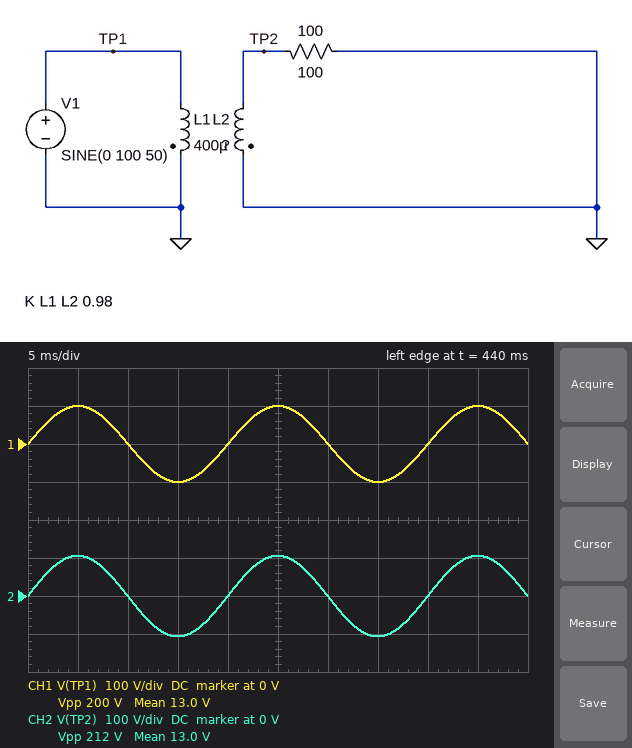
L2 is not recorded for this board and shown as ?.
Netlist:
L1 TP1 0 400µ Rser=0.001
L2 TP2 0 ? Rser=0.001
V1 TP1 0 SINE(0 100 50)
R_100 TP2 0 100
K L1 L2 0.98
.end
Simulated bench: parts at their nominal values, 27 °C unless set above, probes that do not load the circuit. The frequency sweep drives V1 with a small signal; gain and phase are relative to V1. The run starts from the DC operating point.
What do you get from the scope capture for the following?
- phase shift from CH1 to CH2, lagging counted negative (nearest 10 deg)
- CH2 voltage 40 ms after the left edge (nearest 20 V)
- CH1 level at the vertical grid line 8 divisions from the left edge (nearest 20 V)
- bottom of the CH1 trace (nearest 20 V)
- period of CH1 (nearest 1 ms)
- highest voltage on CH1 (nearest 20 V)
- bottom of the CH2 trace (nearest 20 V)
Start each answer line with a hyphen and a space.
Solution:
- 0 deg
- 0 V
- 0 V
- -100 V
- 20 ms
- 100 V
- -100 V
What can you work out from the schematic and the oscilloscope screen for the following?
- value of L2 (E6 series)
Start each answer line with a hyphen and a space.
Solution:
- 470 µH
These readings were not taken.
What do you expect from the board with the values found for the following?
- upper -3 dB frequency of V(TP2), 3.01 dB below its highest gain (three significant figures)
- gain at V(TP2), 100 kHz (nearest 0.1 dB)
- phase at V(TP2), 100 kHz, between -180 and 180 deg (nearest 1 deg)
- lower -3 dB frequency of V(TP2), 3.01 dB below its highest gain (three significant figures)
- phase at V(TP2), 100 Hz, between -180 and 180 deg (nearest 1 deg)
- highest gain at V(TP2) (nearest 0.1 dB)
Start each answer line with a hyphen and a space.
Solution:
- 855 kHz
- 0.5 dB
- -7 deg
- 398 mHz
- 0 deg
- 0.5 dB
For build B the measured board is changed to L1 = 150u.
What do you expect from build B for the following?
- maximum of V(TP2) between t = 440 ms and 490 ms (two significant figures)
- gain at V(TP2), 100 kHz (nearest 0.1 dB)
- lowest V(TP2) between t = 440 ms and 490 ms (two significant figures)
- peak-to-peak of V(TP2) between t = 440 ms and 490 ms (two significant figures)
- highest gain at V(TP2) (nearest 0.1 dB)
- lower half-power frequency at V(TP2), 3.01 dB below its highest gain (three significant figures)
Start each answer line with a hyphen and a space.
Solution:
- 170 V
- 4.7 dB
- -170 V
- 350 V
- 4.8 dB
- 1.06 Hz
